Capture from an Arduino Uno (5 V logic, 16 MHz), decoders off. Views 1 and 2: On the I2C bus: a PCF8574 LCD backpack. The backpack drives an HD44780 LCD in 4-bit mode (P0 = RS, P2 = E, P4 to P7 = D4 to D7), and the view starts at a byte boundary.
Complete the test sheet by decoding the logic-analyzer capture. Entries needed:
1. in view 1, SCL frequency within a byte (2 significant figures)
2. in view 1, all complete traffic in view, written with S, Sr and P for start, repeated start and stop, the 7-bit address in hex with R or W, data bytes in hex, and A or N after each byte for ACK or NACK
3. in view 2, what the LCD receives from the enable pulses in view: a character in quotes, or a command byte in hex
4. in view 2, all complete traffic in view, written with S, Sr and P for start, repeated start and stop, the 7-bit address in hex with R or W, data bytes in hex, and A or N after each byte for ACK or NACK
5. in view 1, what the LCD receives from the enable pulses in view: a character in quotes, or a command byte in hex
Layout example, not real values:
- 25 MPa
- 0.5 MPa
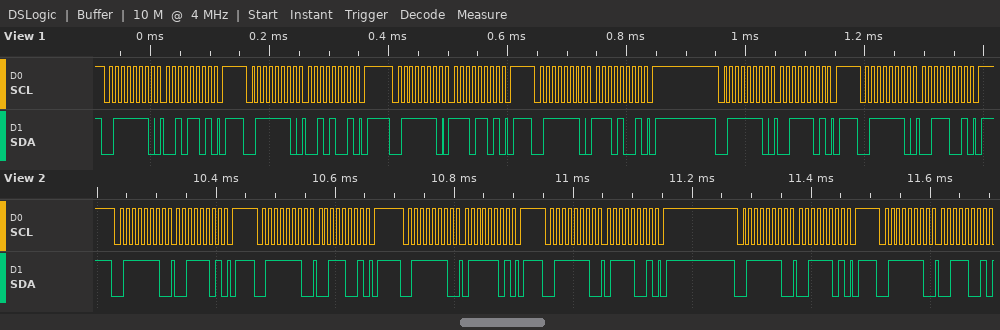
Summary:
- 100 kHz
- S 3FW A 2D A P S 3FW A 29 A P S 3FW A ED A P S 3FW A E9 A P S 3FW A 3D A P S 3FW A 39 A P
- '7'
- S 3FW A 3D A P S 3FW A 39 A P S 3FW A 7D A P S 3FW A 79 A P S 3FW A 3D A P S 3FW A 39 A
- '.'
